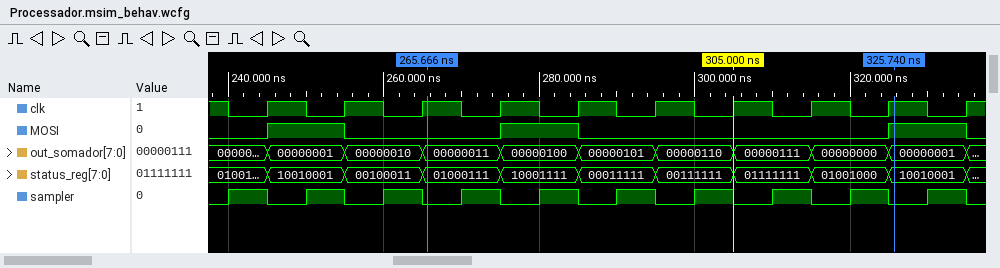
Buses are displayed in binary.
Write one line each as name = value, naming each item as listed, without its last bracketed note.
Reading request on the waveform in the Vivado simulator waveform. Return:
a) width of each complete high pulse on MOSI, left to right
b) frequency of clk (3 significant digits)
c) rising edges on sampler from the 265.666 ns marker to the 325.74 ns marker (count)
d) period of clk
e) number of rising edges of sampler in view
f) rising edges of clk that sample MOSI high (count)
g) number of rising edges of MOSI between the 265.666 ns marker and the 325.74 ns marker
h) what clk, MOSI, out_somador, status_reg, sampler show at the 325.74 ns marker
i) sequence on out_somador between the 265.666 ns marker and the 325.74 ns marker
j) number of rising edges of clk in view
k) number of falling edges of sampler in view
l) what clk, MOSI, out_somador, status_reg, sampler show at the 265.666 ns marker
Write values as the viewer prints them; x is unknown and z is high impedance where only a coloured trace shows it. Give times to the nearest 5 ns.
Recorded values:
width of each complete high pulse on MOSI, left to right = 10 ns, 10 ns, 10 ns
frequency of clk = 100 MHz
rising edges on sampler from the 265.666 ns marker to the 325.74 ns marker = 6
period of clk = 10 ns
number of rising edges of sampler in view = 10
rising edges of clk that sample MOSI high = 3
number of rising edges of MOSI between the 265.666 ns marker and the 325.74 ns marker = 2
what clk, MOSI, out_somador, status_reg, sampler show at the 325.74 ns marker = clk=1, MOSI=1, out_somador=00000001, status_reg=10010001, sampler=0
sequence on out_somador between the 265.666 ns marker and the 325.74 ns marker = 00000011, 00000100, 00000101, 00000110, 00000111, 00000000, 00000001
number of rising edges of clk in view = 10
number of falling edges of sampler in view = 10
what clk, MOSI, out_somador, status_reg, sampler show at the 265.666 ns marker = clk=1, MOSI=0, out_somador=00000011, status_reg=01000111, sampler=0
